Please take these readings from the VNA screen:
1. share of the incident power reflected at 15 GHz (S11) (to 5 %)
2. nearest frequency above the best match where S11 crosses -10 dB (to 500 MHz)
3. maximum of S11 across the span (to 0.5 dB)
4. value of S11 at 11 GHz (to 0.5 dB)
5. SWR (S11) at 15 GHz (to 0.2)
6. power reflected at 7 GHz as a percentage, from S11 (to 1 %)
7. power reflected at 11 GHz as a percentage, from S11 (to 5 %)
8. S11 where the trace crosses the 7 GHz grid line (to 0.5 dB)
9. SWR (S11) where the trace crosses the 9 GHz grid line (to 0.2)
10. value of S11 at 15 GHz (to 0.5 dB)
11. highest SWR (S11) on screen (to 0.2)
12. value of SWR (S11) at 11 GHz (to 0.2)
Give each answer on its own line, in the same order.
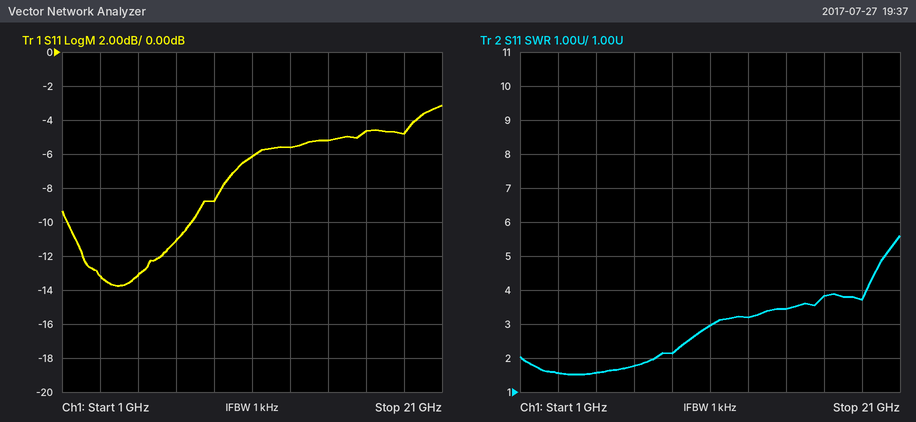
30 %
8.0 GHz
-3.0 dB
-6.0 dB
3.4
8 %
25 %
-11.0 dB
2.2
-5.0 dB
5.6
3.0
